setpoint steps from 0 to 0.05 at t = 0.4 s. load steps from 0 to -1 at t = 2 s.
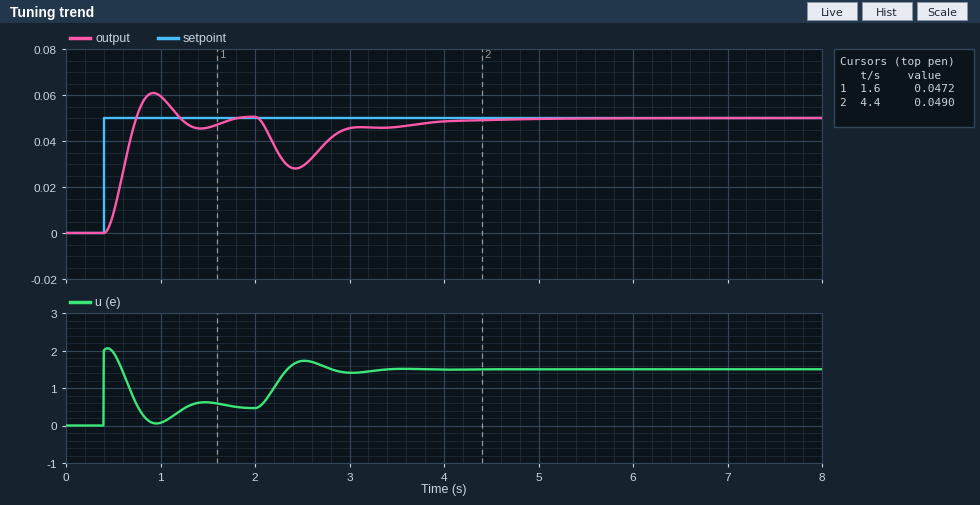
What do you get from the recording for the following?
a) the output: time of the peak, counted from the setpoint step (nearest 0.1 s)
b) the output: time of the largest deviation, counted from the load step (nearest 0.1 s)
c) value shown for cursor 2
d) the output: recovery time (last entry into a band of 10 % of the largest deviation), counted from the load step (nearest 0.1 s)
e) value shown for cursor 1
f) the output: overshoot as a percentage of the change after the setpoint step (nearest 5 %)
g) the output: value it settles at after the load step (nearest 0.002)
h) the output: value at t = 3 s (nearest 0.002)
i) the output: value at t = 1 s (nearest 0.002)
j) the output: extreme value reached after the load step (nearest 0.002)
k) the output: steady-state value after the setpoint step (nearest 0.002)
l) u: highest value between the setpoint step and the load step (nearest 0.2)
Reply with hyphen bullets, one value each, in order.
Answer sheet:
- 0.5 s
- 0.4 s
- 0.0490
- 1.8 s
- 0.0472
- 20 %
- 0.050
- 0.046
- 0.060
- 0.028
- 0.050
- 2.0
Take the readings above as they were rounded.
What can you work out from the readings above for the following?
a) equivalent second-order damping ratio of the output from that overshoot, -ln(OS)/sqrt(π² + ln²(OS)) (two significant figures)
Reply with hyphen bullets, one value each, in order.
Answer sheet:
- 0.46
